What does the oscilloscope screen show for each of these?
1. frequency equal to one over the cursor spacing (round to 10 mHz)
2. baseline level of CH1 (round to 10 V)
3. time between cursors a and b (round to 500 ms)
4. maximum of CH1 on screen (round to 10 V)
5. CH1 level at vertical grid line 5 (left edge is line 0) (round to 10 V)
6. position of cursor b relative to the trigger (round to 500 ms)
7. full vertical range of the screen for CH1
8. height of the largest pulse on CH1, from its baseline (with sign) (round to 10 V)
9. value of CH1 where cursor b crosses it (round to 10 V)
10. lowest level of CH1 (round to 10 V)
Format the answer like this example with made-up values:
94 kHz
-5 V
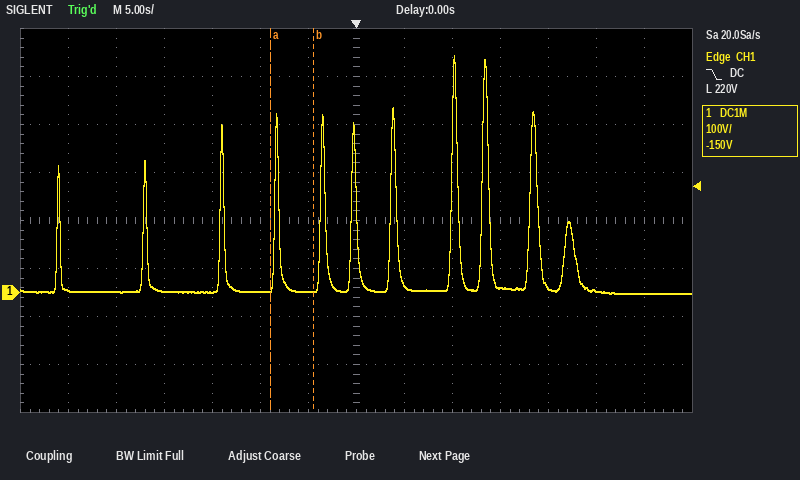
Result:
220 mHz
0 V
4.5 s
490 V
0 V
-4.5 s
800 V
+490 V
0 V
0 V
